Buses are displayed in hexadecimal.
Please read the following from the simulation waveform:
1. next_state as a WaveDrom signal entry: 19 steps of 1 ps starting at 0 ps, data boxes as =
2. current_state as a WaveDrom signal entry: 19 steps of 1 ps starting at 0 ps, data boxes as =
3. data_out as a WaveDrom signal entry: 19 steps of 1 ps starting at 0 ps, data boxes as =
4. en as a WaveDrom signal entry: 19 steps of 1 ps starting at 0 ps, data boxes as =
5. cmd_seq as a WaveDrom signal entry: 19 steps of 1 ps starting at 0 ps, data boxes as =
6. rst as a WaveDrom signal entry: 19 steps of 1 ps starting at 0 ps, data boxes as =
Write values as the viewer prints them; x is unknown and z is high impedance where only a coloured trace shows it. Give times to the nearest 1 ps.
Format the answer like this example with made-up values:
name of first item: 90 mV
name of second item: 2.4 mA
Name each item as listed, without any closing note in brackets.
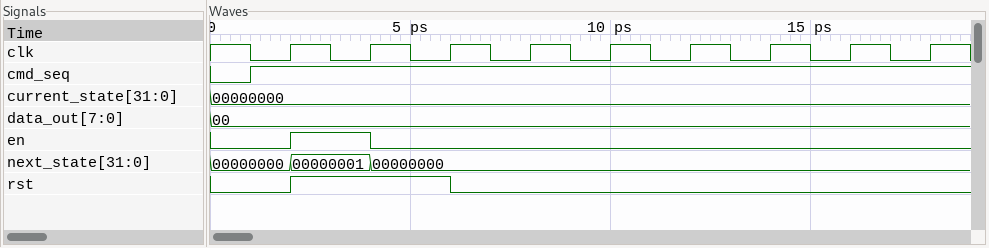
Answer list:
next_state as a WaveDrom signal entry: 19 steps of 1 ps starting at 0 ps, data boxes as =: {name: 'next_state', wave: '=.=.=..............', data: '00000000 00000001 00000000'}
current_state as a WaveDrom signal entry: 19 steps of 1 ps starting at 0 ps, data boxes as =: {name: 'current_state', wave: '=..................', data: '00000000'}
data_out as a WaveDrom signal entry: 19 steps of 1 ps starting at 0 ps, data boxes as =: {name: 'data_out', wave: '=..................', data: '00'}
en as a WaveDrom signal entry: 19 steps of 1 ps starting at 0 ps, data boxes as =: {name: 'en', wave: '0.1.0..............'}
cmd_seq as a WaveDrom signal entry: 19 steps of 1 ps starting at 0 ps, data boxes as =: {name: 'cmd_seq', wave: '01.................'}
rst as a WaveDrom signal entry: 19 steps of 1 ps starting at 0 ps, data boxes as =: {name: 'rst', wave: '0.1...0............'}
